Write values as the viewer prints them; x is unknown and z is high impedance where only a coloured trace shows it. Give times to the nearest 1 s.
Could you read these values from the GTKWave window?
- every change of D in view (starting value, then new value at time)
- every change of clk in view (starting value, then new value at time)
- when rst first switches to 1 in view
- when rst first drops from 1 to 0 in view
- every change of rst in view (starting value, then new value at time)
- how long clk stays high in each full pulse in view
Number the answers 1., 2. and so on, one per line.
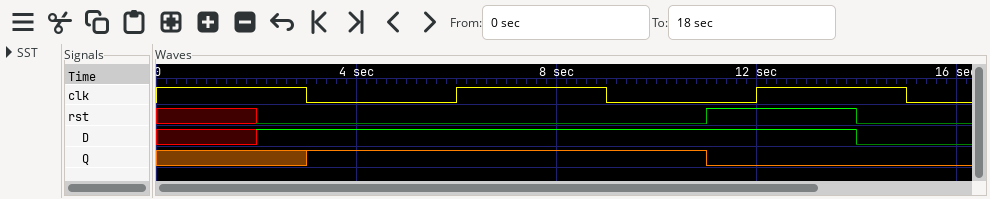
1. x, 1 at 2 s, 0 at 14 s
2. 1, 0 at 3 s, 1 at 6 s, 0 at 9 s, 1 at 12 s, 0 at 15 s
3. 11 s
4. 14 s
5. x, 0 at 2 s, 1 at 11 s, 0 at 14 s
6. 3 s, 3 s
